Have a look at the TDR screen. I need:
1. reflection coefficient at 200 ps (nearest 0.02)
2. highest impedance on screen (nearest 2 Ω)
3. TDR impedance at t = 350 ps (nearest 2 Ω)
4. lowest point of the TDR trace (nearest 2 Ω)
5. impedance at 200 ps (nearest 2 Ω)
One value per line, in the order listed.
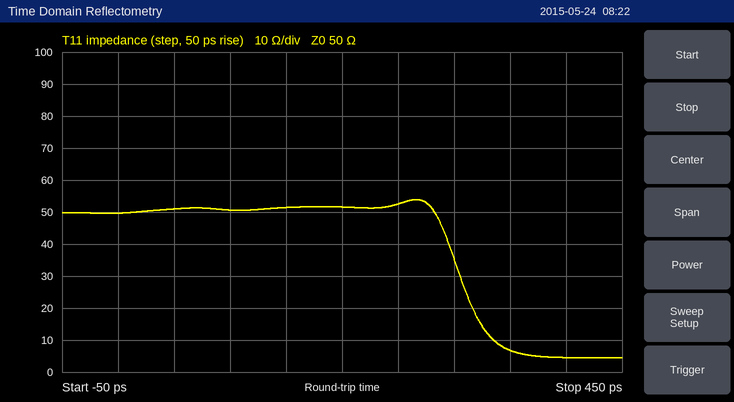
+0.02
54 Ω
6 Ω
4 Ω
52 Ω
